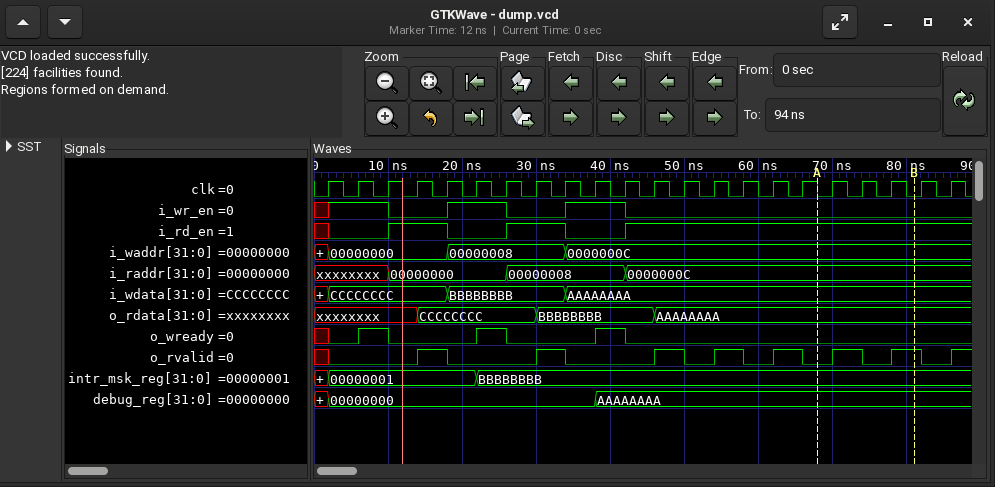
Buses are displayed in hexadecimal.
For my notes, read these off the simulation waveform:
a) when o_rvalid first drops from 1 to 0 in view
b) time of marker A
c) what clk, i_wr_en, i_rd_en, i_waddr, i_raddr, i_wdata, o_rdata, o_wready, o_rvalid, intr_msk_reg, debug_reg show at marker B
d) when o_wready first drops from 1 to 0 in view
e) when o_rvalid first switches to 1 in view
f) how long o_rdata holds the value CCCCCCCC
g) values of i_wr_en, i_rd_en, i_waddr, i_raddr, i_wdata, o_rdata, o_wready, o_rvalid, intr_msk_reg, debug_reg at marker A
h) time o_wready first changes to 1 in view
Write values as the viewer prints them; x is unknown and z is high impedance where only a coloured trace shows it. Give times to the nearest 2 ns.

18 ns
68 ns
clk=0, i_wr_en=0, i_rd_en=1, i_waddr=0000000C, i_raddr=0000000C, i_wdata=AAAAAAAA, o_rdata=AAAAAAAA, o_wready=0, o_rvalid=1, intr_msk_reg=BBBBBBBB, debug_reg=AAAAAAAA
10 ns
14 ns
16 ns
i_wr_en=0, i_rd_en=1, i_waddr=0000000C, i_raddr=0000000C, i_wdata=AAAAAAAA, o_rdata=AAAAAAAA, o_wready=0, o_rvalid=0, intr_msk_reg=BBBBBBBB, debug_reg=AAAAAAAA
6 ns
